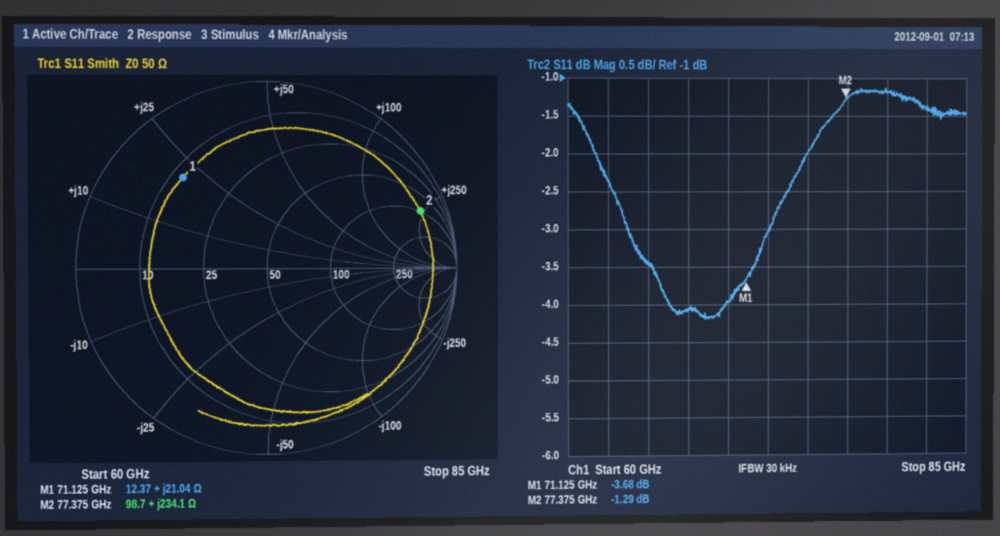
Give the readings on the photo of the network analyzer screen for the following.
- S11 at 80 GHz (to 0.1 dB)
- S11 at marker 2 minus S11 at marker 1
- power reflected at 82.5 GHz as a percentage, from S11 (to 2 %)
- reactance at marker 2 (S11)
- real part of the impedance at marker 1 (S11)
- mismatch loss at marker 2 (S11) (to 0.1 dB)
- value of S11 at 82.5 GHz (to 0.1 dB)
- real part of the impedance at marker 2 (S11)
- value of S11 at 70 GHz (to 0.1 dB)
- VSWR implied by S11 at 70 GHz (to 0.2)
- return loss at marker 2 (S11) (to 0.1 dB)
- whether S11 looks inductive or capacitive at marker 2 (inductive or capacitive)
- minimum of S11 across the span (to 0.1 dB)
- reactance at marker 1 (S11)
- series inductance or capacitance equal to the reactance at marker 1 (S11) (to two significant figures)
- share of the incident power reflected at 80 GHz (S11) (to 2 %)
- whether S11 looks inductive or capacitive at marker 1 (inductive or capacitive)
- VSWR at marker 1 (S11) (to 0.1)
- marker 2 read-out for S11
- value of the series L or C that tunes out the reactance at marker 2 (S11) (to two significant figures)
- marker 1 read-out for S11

-1.2 dB
2.39 dB
72 %
+234.1 Ω
12.37 Ω
5.9 dB
-1.4 dB
98.7 Ω
-4.0 dB
4.4
1.3 dB
inductive
-4.2 dB
+21.04 Ω
47 pH
76 %
inductive
4.8
-1.29 dB
8.8 fF
-3.68 dB
